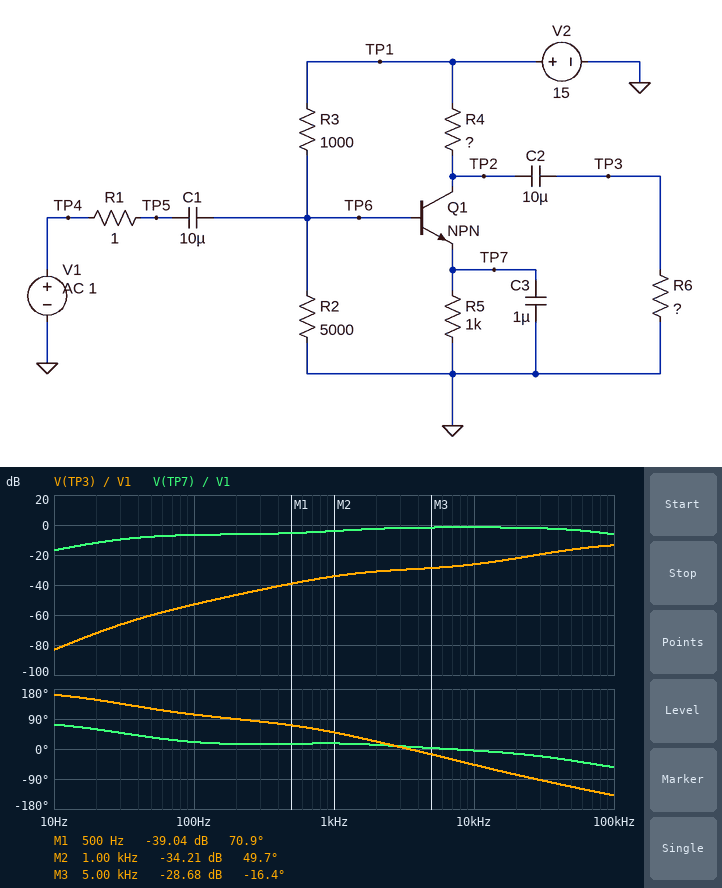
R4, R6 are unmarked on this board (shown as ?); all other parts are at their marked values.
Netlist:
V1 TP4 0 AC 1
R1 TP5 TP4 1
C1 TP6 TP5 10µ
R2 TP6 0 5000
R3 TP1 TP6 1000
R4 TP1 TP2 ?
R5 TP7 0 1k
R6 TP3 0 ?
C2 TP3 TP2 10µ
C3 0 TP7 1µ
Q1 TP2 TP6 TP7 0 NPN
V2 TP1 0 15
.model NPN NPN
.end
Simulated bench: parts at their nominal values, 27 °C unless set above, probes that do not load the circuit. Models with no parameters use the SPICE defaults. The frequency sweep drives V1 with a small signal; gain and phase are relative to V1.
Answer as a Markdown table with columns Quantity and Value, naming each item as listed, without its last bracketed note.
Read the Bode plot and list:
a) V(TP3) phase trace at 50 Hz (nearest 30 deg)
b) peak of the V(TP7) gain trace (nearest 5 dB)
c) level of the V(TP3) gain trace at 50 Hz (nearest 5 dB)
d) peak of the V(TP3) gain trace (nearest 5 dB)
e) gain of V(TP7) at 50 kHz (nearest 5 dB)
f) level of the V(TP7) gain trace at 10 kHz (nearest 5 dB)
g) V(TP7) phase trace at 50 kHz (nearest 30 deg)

| Quantity | Value |
|---|---|
| V(TP3) phase trace at 50 Hz | 120 deg |
| peak of the V(TP7) gain trace | 0 dB |
| level of the V(TP3) gain trace at 50 Hz | -60 dB |
| peak of the V(TP3) gain trace | -15 dB |
| gain of V(TP7) at 50 kHz | -5 dB |
| level of the V(TP7) gain trace at 10 kHz | 0 dB |
| V(TP7) phase trace at 50 kHz | -30 deg |
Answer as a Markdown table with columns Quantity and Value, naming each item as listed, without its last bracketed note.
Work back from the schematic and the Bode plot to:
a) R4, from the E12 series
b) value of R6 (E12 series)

| Quantity | Value |
|---|---|
| R4, from the E12 series | 470 Ω |
| value of R6 | 0.82 Ω |
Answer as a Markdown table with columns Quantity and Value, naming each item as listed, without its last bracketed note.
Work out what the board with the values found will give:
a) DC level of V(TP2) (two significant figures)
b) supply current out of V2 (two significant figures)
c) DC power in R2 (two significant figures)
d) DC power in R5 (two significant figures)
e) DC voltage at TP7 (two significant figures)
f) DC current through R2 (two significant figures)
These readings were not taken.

| Quantity | Value |
|---|---|
| DC level of V(TP2) | 11 V |
| supply current out of V2 | 13 mA |
| DC power in R2 | 26 mW |
| DC power in R5 | 110 mW |
| DC voltage at TP7 | 11 V |
| DC current through R2 | 2.3 mA |
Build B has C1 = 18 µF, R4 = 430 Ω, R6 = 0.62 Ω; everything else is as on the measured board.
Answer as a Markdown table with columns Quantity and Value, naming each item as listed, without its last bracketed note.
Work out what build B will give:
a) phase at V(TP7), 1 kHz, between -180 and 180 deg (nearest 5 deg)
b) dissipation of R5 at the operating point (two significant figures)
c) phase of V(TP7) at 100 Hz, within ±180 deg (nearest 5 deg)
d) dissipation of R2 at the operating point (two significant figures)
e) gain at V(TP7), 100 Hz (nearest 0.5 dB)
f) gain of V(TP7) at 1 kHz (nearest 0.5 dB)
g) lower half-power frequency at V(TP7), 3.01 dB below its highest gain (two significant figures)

| Quantity | Value |
|---|---|
| phase at V(TP7), 1 kHz, between -180 and 180 deg | 10 deg |
| dissipation of R5 at the operating point | 120 mW |
| phase of V(TP7) at 100 Hz, within ±180 deg | 15 deg |
| dissipation of R2 at the operating point | 27 mW |
| gain at V(TP7), 100 Hz | -4.0 dB |
| gain of V(TP7) at 1 kHz | -2.0 dB |
| lower half-power frequency at V(TP7), 3.01 dB below its highest gain | 82 Hz |
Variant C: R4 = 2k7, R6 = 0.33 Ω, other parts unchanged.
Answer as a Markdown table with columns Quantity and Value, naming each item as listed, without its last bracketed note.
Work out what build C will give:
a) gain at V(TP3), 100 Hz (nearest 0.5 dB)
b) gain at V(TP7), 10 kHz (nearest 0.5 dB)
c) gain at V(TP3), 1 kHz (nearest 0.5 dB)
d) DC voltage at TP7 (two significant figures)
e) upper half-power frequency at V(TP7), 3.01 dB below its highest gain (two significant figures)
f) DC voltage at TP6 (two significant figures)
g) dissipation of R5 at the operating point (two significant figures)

| Quantity | Value |
|---|---|
| gain at V(TP3), 100 Hz | -60.5 dB |
| gain at V(TP7), 10 kHz | -6.0 dB |
| gain at V(TP3), 1 kHz | -40.5 dB |
| DC voltage at TP7 | 7.6 V |
| upper half-power frequency at V(TP7), 3.01 dB below its highest gain | 78 kHz |
| DC voltage at TP6 | 8.4 V |
| dissipation of R5 at the operating point | 58 mW |
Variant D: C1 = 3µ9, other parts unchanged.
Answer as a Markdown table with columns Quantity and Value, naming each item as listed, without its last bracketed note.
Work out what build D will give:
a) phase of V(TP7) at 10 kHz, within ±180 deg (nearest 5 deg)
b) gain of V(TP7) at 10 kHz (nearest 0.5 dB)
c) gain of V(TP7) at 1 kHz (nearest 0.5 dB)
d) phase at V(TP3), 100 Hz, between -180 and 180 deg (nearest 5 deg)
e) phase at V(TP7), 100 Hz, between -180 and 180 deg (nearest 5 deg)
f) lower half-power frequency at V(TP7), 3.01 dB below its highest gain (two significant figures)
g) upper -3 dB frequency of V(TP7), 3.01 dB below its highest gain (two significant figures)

| Quantity | Value |
|---|---|
| phase of V(TP7) at 10 kHz, within ±180 deg | 0 deg |
| gain of V(TP7) at 10 kHz | -2.0 dB |
| gain of V(TP7) at 1 kHz | -8.0 dB |
| phase at V(TP3), 100 Hz, between -180 and 180 deg | 110 deg |
| phase at V(TP7), 100 Hz, between -180 and 180 deg | 30 deg |
| lower half-power frequency at V(TP7), 3.01 dB below its highest gain | 2.1 kHz |
| upper -3 dB frequency of V(TP7), 3.01 dB below its highest gain | 75 kHz |
